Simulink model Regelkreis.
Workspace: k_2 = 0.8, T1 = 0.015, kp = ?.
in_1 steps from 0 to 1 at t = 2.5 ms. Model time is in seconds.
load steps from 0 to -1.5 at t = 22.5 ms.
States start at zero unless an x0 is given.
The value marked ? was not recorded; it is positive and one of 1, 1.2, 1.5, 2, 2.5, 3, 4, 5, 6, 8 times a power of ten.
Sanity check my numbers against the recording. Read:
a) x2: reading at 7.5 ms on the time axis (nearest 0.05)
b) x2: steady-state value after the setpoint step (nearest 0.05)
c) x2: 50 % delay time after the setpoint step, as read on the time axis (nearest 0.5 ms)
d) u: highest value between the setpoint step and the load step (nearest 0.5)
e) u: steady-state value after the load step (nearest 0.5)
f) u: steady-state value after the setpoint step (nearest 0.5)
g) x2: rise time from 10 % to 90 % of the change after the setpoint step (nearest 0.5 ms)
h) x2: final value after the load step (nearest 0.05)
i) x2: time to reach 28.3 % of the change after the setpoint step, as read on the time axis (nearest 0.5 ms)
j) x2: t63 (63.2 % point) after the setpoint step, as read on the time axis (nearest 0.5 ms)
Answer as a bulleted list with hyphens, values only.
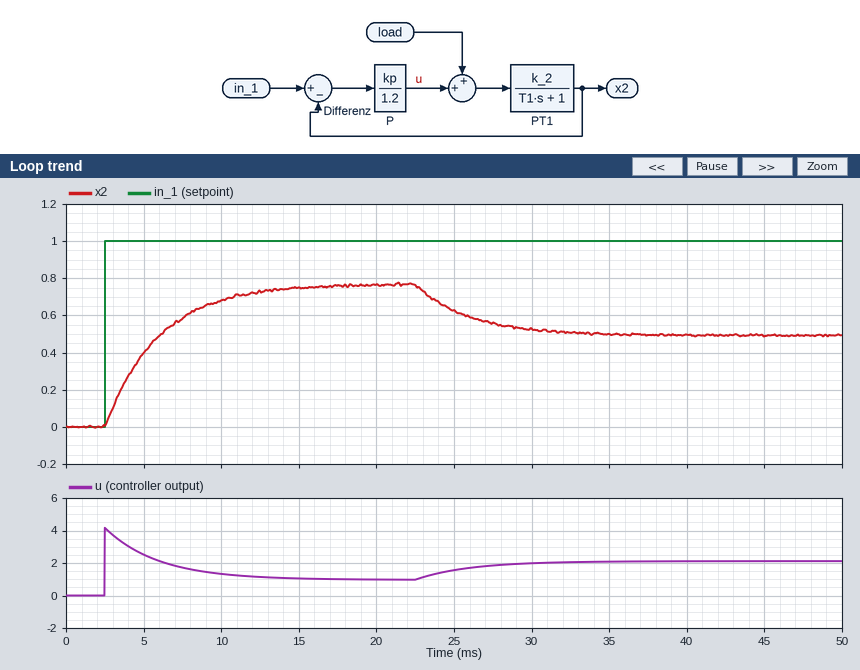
- 0.60
- 0.75
- 5.0 ms
- 4.0
- 2.0
- 1.0
- 7.5 ms
- 0.50
- 3.5 ms
- 6.0 ms
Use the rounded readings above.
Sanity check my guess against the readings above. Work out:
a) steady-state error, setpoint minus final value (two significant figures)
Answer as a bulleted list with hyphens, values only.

- 0.25
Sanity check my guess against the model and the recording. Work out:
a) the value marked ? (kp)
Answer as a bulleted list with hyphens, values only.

- 5
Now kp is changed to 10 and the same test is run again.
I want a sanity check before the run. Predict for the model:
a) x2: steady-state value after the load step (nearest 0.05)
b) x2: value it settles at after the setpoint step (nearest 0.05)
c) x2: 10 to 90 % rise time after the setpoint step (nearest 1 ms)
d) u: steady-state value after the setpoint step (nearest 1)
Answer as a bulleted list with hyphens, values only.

- 0.70
- 0.85
- 4 ms
- 1
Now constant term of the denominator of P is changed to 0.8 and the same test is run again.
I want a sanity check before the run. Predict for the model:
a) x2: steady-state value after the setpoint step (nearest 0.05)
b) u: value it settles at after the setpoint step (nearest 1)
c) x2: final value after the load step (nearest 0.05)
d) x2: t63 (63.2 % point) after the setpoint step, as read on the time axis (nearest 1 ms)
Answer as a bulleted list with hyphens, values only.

- 0.85
- 1
- 0.65
- 5 ms
